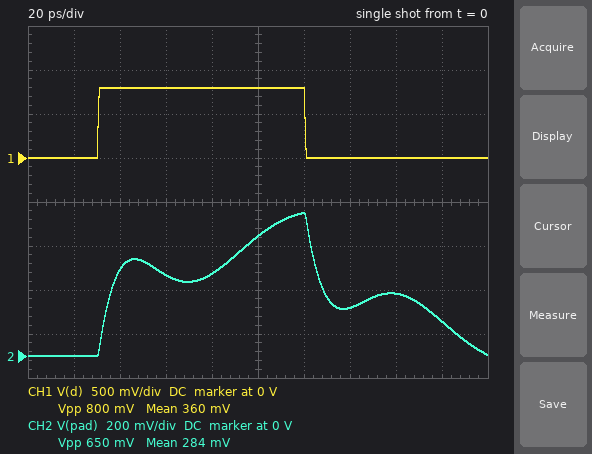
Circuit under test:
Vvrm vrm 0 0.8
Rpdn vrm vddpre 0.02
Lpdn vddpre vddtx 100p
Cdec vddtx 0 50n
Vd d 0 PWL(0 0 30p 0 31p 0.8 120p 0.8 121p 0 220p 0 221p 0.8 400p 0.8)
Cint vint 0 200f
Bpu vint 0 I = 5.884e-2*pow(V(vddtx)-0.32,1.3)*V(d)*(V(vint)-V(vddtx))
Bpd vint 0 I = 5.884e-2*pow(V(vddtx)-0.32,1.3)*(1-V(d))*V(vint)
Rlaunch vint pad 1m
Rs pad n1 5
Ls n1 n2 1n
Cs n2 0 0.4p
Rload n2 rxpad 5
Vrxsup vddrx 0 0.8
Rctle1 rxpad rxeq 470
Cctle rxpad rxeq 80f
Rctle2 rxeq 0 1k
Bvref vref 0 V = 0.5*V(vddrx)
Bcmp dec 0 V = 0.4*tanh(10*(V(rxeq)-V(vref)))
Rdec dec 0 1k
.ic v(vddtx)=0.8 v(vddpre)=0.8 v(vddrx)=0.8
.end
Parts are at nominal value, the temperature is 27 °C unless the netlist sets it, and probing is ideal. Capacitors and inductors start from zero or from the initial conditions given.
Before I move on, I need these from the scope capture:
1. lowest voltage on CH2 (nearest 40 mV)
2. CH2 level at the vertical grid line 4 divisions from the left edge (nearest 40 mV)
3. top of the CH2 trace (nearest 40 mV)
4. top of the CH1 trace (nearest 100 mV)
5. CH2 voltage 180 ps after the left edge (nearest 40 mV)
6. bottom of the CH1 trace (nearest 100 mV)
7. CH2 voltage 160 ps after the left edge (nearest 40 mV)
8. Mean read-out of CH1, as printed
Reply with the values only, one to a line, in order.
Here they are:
0 V
360 mV
640 mV
800 mV
160 mV
0 V
280 mV
360 mV
